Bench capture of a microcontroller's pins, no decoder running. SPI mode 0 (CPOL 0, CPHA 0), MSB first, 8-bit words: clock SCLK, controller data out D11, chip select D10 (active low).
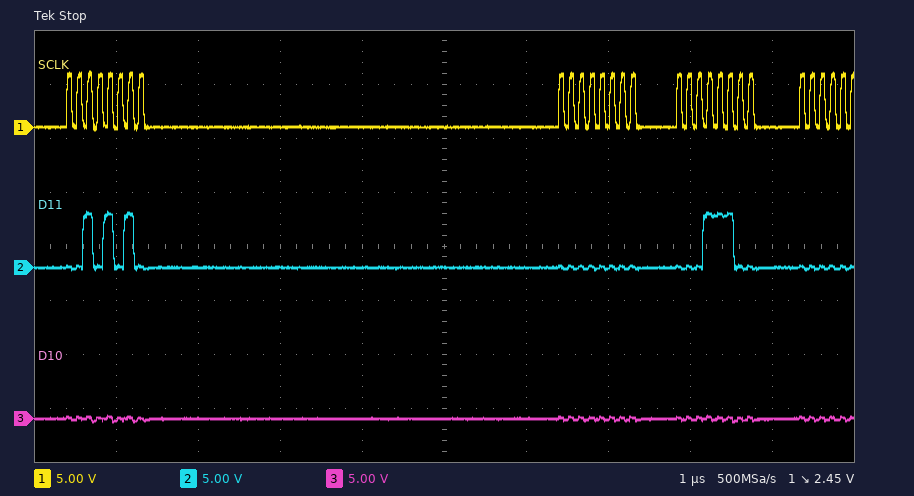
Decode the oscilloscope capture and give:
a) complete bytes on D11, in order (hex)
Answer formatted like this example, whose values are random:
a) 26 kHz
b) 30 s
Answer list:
a) 2A 00 1C
